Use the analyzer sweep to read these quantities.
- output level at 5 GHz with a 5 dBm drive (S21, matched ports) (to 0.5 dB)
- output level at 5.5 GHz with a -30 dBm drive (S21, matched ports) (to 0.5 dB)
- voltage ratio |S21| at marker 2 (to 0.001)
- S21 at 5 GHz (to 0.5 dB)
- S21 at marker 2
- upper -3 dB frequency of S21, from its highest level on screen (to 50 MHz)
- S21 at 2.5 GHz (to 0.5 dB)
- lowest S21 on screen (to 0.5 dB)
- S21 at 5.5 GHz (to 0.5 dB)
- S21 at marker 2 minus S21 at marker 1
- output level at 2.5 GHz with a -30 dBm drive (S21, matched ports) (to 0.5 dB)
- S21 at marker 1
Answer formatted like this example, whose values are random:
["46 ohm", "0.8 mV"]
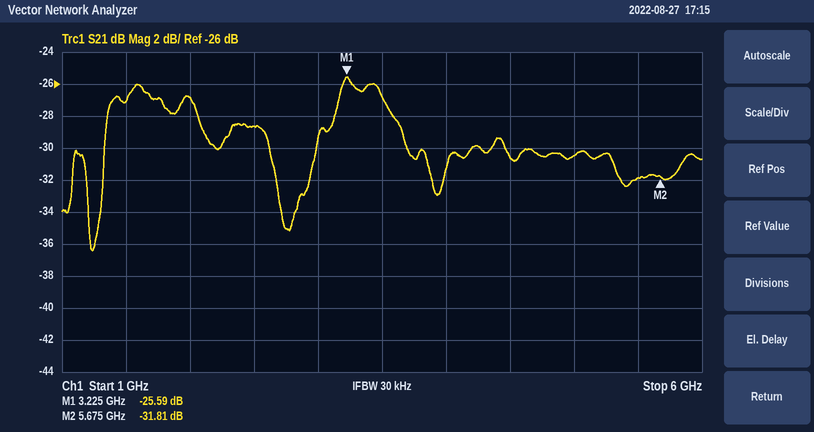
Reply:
["-25.5 dBm", "-62.0 dBm", "0.026", "-30.5 dB", "-31.81 dB", "3.65 GHz", "-28.5 dB", "-36.5 dB", "-32.0 dB", "-6.22 dB", "-58.5 dBm", "-25.59 dB"]
